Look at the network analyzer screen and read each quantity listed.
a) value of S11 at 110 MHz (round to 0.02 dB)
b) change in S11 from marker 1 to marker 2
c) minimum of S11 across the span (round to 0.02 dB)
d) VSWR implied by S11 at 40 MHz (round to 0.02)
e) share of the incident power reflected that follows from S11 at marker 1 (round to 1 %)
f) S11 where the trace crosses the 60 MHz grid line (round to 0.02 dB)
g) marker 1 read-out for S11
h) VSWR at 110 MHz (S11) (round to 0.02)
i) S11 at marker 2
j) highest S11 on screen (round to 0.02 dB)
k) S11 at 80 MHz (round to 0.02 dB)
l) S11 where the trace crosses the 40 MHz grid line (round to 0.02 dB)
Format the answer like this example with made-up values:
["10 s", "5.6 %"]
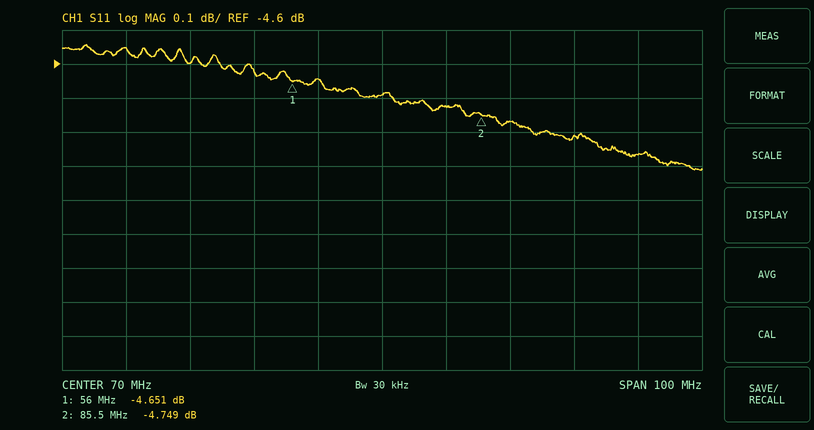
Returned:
["-4.86 dB", "-0.098 dB", "-4.92 dB", "3.86", "34 %", "-4.64 dB", "-4.651 dB", "3.66", "-4.749 dB", "-4.54 dB", "-4.72 dB", "-4.60 dB"]
